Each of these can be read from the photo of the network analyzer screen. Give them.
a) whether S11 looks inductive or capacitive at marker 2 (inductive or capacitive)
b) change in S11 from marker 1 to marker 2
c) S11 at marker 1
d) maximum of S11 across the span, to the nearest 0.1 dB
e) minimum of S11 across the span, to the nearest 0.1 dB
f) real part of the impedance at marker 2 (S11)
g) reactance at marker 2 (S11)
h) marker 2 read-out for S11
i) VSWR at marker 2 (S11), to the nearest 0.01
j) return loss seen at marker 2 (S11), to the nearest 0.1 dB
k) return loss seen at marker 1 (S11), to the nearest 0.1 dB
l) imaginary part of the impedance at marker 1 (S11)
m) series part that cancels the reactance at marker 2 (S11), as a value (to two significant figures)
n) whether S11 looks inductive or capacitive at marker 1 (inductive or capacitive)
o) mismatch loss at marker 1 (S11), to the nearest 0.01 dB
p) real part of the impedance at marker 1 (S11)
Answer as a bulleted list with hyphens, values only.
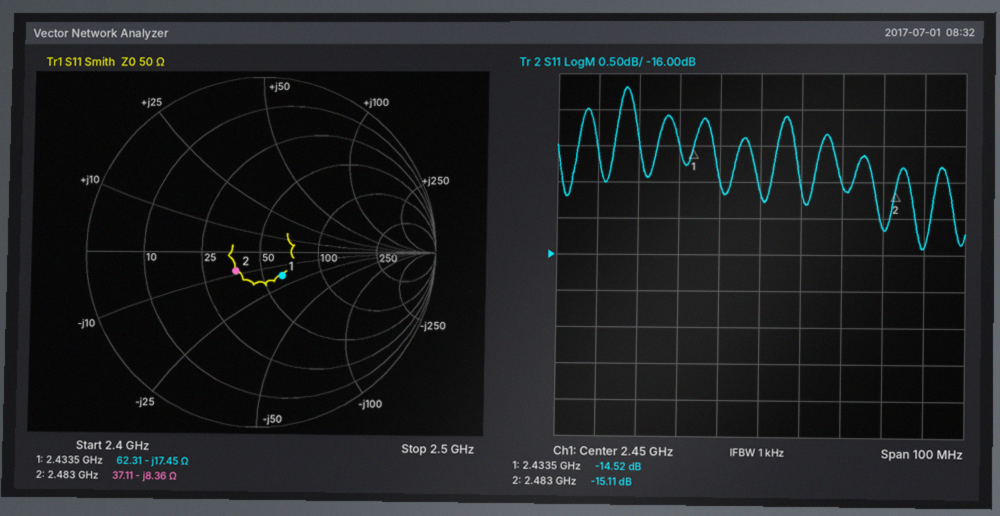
- capacitive
- -0.59 dB
- -14.52 dB
- -13.7 dB
- -15.9 dB
- 37.11 Ω
- -8.36 Ω
- -15.11 dB
- 1.43
- 15.1 dB
- 14.5 dB
- -17.45 Ω
- 540 pH
- capacitive
- 0.16 dB
- 62.31 Ω
